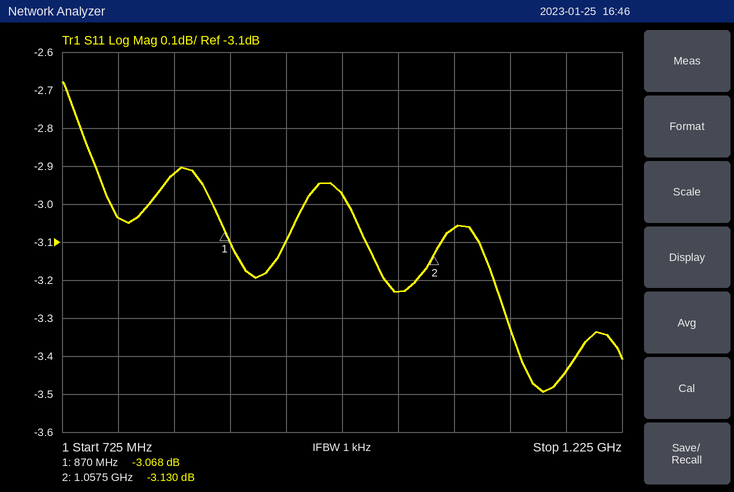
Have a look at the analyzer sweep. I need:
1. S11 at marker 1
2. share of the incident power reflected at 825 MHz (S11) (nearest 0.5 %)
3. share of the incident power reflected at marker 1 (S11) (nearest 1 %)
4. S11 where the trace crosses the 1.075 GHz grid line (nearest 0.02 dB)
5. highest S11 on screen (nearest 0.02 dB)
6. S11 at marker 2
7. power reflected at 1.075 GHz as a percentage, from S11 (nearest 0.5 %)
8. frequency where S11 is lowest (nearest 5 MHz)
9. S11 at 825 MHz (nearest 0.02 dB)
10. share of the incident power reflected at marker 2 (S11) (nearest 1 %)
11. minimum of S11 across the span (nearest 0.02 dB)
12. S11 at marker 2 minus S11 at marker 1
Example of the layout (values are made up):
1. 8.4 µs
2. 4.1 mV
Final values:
1. -3.068 dB
2. 51.0 %
3. 49 %
4. -3.06 dB
5. -2.68 dB
6. -3.130 dB
7. 49.5 %
8. 1.155 GHz
9. -2.92 dB
10. 49 %
11. -3.50 dB
12. -0.062 dB
